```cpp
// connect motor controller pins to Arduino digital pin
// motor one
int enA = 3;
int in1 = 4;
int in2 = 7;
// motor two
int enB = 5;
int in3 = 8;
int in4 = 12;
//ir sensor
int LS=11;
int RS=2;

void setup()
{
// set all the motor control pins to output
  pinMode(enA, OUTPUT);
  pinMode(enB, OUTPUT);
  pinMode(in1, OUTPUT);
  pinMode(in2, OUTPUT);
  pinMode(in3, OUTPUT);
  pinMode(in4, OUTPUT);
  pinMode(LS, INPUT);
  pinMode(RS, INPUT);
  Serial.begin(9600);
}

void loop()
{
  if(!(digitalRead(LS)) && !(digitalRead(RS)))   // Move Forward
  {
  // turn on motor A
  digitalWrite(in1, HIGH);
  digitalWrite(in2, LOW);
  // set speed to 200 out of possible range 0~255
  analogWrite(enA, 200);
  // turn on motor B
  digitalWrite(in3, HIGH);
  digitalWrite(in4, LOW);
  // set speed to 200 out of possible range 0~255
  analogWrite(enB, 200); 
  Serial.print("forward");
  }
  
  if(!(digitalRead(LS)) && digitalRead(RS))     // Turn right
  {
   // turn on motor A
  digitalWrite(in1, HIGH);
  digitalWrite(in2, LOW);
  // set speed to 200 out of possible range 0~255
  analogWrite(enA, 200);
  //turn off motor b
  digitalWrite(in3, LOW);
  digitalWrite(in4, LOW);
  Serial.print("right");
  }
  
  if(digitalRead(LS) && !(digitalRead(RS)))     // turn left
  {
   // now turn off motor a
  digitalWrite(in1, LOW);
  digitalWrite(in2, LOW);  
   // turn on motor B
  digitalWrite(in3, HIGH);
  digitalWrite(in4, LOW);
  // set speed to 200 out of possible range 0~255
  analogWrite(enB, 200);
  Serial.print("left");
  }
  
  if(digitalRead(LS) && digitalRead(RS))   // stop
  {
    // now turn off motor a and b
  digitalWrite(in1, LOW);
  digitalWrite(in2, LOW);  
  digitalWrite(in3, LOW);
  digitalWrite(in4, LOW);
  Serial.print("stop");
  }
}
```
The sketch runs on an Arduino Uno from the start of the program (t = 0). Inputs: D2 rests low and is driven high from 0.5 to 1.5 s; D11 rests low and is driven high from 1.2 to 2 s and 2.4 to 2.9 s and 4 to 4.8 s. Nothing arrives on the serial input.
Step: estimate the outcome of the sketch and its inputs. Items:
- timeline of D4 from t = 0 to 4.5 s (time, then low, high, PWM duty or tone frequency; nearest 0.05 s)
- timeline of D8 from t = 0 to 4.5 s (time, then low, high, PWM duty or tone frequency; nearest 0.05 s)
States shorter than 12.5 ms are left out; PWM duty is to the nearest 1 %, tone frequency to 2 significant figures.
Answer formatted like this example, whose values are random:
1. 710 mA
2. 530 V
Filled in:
1. 0 s high; 1.2 s low; 2 s high; 2.4 s low; 2.9 s high; 4 s low
2. 0 s high; 0.5 s low; 1.5 s high
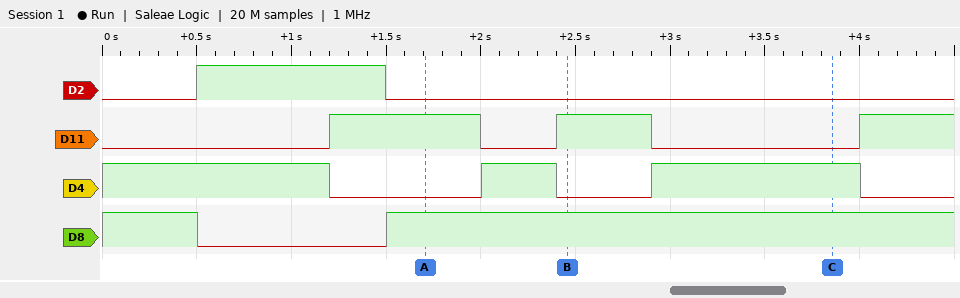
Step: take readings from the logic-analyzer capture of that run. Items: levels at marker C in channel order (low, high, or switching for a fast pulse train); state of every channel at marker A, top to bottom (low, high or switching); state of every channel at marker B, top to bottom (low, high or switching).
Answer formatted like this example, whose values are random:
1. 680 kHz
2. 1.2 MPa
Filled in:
1. D2 low, D11 low, D4 high, D8 high
2. D2 low, D11 high, D4 low, D8 high
3. D2 low, D11 high, D4 low, D8 high
